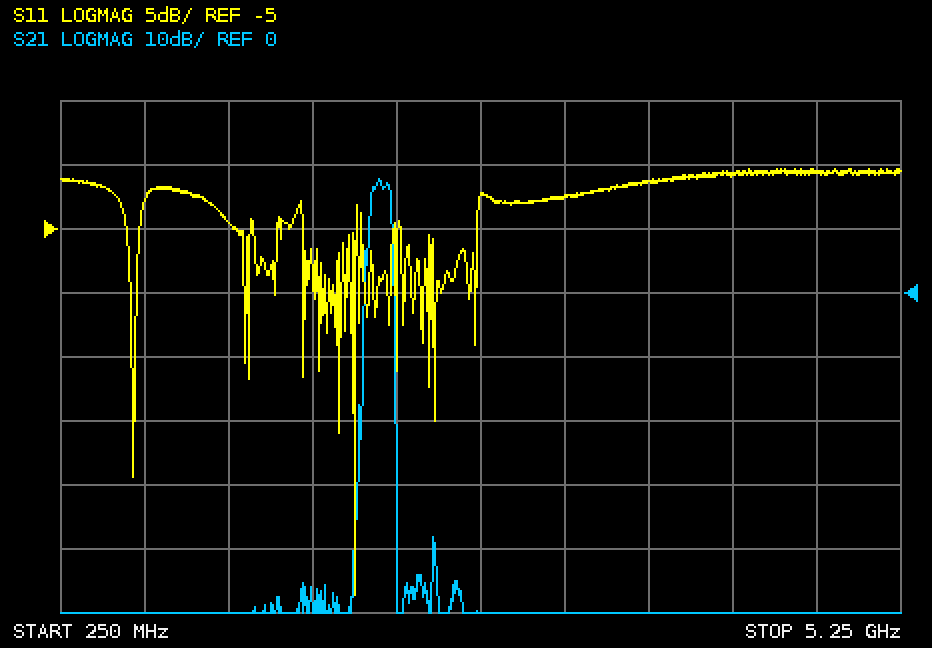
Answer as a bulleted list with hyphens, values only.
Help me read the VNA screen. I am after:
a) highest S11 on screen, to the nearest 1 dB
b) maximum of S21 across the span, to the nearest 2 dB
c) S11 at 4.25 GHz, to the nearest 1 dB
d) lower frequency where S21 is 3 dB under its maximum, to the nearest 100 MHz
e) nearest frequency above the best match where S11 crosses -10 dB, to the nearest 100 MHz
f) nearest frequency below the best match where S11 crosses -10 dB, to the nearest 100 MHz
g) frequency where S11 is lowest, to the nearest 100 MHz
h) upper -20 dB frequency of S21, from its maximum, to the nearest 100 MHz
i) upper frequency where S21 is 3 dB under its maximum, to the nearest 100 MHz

- 0 dB
- 18 dB
- -1 dB
- 2.1 GHz
- 2.0 GHz
- 2.0 GHz
- 2.0 GHz
- 2.2 GHz
- 2.2 GHz
